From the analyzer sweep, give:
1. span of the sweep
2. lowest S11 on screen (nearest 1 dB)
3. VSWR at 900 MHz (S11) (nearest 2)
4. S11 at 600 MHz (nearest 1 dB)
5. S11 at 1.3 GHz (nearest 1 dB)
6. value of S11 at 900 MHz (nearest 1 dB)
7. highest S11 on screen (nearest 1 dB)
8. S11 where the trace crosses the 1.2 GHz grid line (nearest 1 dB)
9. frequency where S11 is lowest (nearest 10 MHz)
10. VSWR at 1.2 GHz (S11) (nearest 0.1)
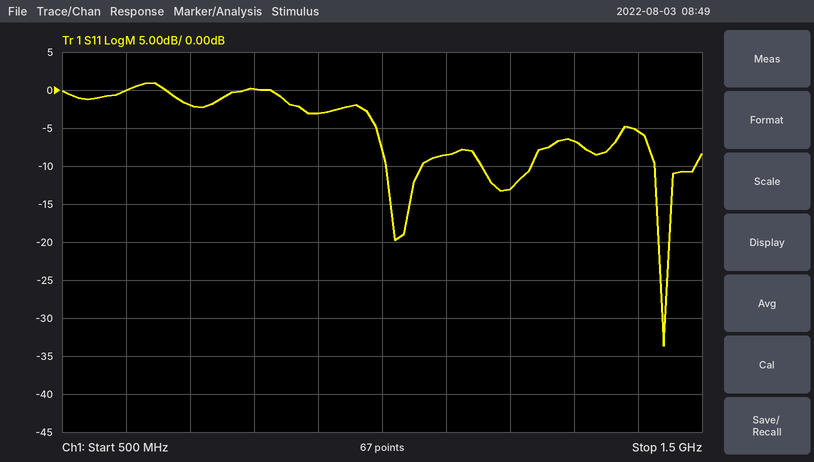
1 GHz
-34 dB
6
0 dB
-7 dB
-3 dB
1 dB
-13 dB
1.44 GHz
1.6
